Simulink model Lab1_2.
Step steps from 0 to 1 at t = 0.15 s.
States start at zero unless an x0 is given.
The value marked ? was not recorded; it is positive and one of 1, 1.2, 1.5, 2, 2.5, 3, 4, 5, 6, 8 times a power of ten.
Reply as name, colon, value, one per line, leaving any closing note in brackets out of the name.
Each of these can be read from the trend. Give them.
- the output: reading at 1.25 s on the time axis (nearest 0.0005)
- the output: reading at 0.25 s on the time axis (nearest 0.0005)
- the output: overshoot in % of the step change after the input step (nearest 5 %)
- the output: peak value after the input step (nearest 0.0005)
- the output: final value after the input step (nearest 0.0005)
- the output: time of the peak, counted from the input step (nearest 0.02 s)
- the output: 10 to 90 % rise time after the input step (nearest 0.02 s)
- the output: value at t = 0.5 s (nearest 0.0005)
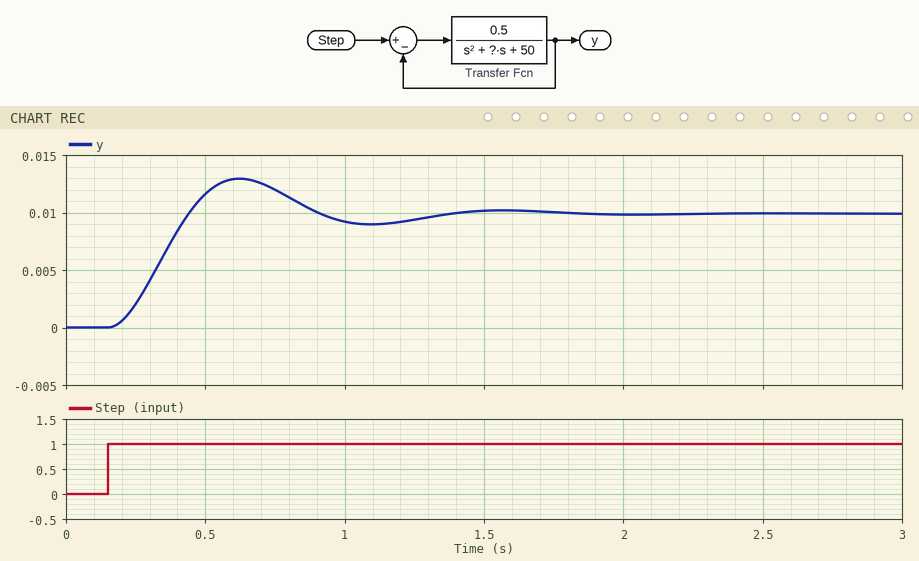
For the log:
the output: reading at 1.25 s on the time axis: 0.0095
the output: reading at 0.25 s on the time axis: 0.0020
the output: overshoot in % of the step change after the input step: 30 %
the output: peak value after the input step: 0.0130
the output: final value after the input step: 0.0100
the output: time of the peak, counted from the input step: 0.48 s
the output: 10 to 90 % rise time after the input step: 0.20 s
the output: value at t = 0.5 s: 0.0115
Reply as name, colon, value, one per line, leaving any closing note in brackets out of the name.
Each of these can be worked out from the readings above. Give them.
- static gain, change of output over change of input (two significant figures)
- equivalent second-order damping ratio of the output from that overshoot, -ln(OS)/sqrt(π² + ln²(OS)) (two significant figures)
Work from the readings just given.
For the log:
static gain, change of output over change of input: 0.010
equivalent second-order damping ratio of the output from that overshoot, -ln(OS)/sqrt(π² + ln²(OS)): 0.36
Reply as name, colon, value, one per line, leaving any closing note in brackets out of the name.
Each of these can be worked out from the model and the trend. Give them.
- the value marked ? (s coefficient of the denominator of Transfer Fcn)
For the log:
the value marked ?: 5
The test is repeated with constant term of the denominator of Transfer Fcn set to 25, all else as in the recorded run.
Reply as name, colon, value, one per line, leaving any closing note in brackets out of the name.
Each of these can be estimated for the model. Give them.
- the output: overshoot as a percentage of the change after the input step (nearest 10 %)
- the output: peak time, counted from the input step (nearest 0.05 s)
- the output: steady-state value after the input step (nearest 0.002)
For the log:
the output: overshoot as a percentage of the change after the input step: 20 %
the output: peak time, counted from the input step: 0.70 s
the output: steady-state value after the input step: 0.020
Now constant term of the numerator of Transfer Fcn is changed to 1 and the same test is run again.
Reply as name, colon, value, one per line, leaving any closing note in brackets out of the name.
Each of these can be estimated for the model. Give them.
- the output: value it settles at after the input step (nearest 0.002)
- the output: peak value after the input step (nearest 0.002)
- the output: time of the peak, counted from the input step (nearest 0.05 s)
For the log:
the output: value it settles at after the input step: 0.020
the output: peak value after the input step: 0.026
the output: time of the peak, counted from the input step: 0.45 s
